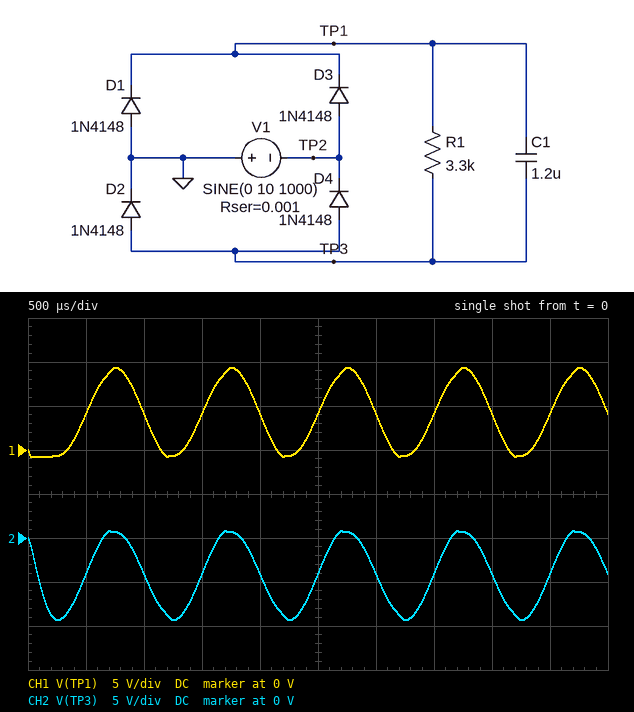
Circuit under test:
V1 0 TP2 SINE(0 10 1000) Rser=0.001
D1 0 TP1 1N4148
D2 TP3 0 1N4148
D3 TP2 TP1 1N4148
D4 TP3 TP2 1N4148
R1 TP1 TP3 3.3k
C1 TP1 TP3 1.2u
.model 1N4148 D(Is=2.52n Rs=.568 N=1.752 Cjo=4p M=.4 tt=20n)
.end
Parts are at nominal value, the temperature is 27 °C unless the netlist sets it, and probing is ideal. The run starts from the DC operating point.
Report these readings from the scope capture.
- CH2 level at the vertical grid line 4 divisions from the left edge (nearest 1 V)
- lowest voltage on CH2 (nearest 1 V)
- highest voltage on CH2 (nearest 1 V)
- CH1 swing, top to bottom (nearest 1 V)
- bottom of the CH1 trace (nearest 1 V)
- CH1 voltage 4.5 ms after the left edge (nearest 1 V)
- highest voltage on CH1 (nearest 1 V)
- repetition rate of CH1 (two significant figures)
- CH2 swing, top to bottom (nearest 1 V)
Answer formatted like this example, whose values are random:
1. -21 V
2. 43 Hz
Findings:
1. -4 V
2. -9 V
3. 1 V
4. 10 V
5. -1 V
6. 4 V
7. 9 V
8. 1.0 kHz
9. 10 V
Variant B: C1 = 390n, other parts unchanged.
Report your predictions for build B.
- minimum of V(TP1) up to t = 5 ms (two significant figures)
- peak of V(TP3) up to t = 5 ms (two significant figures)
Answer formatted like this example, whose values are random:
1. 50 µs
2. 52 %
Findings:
1. -740 mV
2. 720 mV
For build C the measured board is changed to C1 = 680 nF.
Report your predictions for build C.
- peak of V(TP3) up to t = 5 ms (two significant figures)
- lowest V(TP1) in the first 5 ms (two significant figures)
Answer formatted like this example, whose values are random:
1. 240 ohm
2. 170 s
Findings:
1. 730 mV
2. -780 mV
